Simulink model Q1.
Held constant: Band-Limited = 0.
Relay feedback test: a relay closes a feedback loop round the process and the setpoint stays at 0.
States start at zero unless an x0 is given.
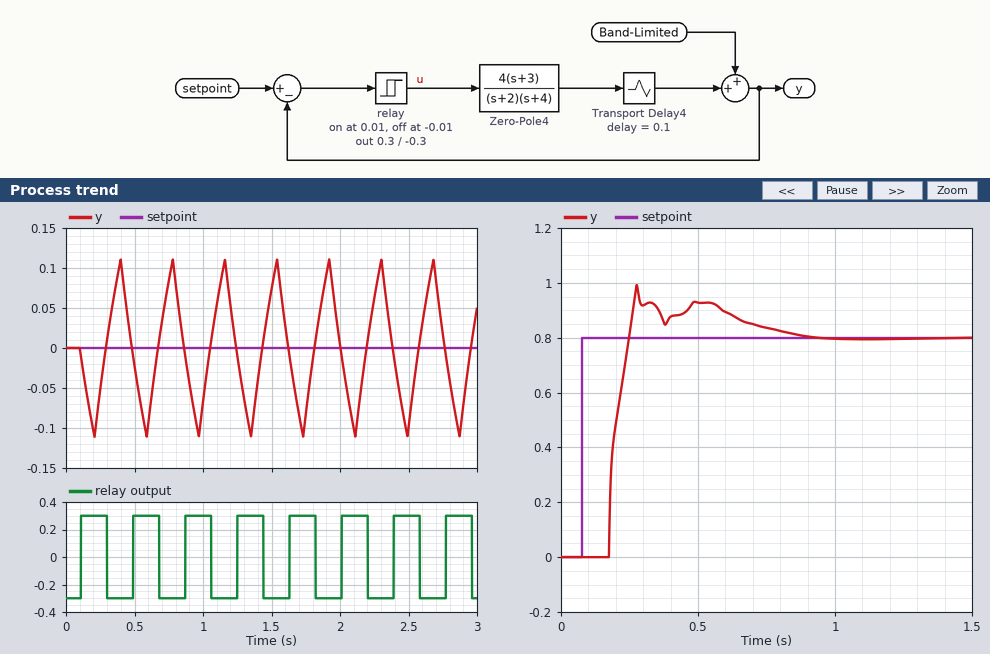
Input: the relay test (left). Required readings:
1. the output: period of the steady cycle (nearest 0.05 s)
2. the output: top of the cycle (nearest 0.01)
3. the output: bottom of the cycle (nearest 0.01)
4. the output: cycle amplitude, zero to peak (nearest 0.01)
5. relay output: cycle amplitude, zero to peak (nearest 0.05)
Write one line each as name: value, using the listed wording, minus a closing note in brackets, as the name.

the output: period of the steady cycle: 0.40 s
the output: top of the cycle: 0.11
the output: bottom of the cycle: -0.11
the output: cycle amplitude, zero to peak: 0.11
relay output: cycle amplitude, zero to peak: 0.30
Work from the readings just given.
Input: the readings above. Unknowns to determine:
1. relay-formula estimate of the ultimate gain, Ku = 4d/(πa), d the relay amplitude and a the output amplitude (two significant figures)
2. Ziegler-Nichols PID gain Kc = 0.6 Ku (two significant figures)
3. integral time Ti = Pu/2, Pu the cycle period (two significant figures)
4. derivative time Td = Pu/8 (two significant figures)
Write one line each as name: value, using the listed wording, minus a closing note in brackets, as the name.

relay-formula estimate of the ultimate gain, Ku = 4d/(πa), d the relay amplitude and a the output amplitude: 3.5
Ziegler-Nichols PID gain Kc = 0.6 Ku: 2.1
integral time Ti = Pu/2, Pu the cycle period: 0.20 s
derivative time Td = Pu/8: 0.050 s
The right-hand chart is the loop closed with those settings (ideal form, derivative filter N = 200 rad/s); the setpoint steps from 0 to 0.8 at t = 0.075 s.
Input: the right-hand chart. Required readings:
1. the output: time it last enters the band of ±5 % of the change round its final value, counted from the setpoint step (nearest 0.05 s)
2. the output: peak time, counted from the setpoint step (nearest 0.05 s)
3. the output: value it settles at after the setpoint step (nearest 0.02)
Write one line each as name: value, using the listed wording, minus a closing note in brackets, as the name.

the output: time it last enters the band of ±5 % of the change round its final value, counted from the setpoint step: 0.65 s
the output: peak time, counted from the setpoint step: 0.20 s
the output: value it settles at after the setpoint step: 0.80
